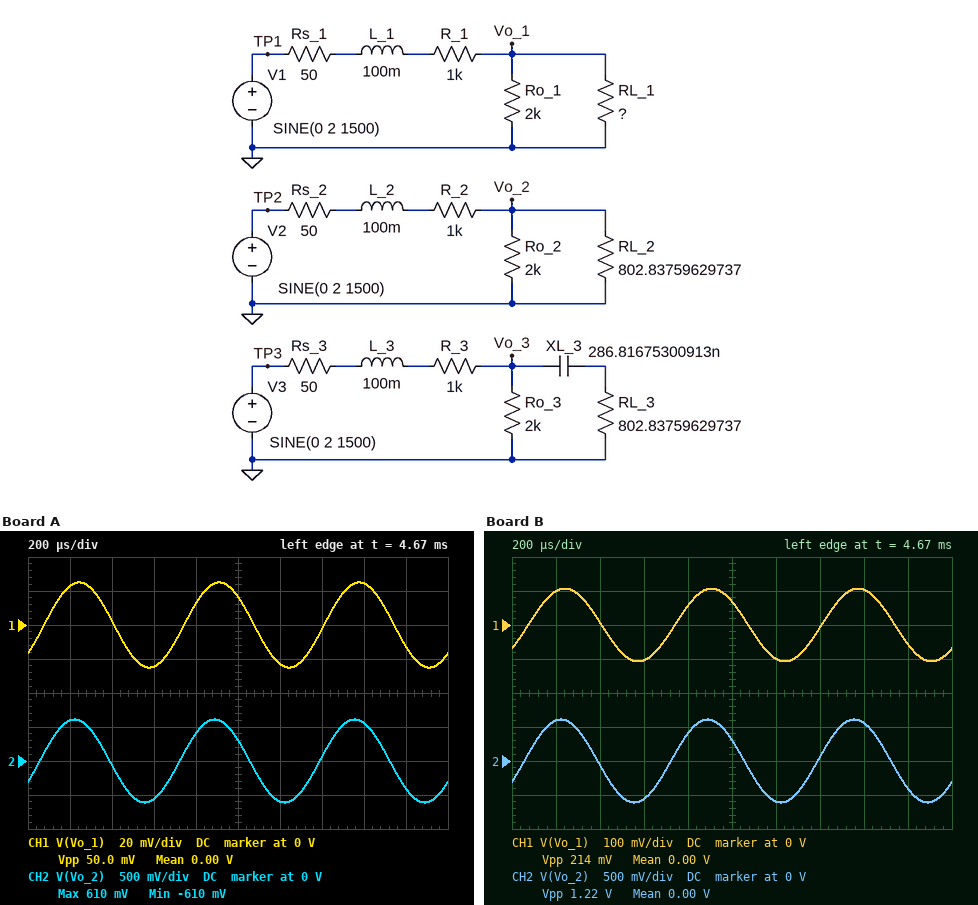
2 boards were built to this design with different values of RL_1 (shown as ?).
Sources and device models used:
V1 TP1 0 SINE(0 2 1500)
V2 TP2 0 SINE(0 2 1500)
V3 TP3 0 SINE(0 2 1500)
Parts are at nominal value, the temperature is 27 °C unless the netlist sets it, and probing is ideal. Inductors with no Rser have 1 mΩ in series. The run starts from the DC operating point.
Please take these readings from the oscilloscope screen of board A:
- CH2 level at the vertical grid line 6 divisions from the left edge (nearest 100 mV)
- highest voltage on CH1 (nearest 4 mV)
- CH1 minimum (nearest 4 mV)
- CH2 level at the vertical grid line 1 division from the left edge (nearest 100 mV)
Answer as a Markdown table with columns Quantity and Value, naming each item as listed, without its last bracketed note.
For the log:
| Quantity | Value |
|---|---|
| CH2 level at the vertical grid line 6 divisions from the left edge | -600 mV |
| highest voltage on CH1 | 24 mV |
| CH1 minimum | -24 mV |
| CH2 level at the vertical grid line 1 division from the left edge | 600 mV |
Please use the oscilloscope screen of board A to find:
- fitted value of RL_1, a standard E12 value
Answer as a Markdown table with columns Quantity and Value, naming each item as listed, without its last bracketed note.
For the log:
| Quantity | Value |
|---|---|
| fitted value of RL_1, a standard E12 value | 18 Ω |
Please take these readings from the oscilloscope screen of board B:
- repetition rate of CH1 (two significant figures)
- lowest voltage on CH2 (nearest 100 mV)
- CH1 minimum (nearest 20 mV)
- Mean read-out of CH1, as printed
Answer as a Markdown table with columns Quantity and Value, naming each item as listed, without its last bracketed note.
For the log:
| Quantity | Value |
|---|---|
| repetition rate of CH1 | 1.5 kHz |
| lowest voltage on CH2 | -600 mV |
| CH1 minimum | -100 mV |
| Mean read-out of CH1, as printed | 0.00 V |
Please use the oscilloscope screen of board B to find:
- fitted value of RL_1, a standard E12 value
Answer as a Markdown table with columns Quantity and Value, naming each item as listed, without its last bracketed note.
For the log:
| Quantity | Value |
|---|---|
| fitted value of RL_1, a standard E12 value | 82 Ω |
